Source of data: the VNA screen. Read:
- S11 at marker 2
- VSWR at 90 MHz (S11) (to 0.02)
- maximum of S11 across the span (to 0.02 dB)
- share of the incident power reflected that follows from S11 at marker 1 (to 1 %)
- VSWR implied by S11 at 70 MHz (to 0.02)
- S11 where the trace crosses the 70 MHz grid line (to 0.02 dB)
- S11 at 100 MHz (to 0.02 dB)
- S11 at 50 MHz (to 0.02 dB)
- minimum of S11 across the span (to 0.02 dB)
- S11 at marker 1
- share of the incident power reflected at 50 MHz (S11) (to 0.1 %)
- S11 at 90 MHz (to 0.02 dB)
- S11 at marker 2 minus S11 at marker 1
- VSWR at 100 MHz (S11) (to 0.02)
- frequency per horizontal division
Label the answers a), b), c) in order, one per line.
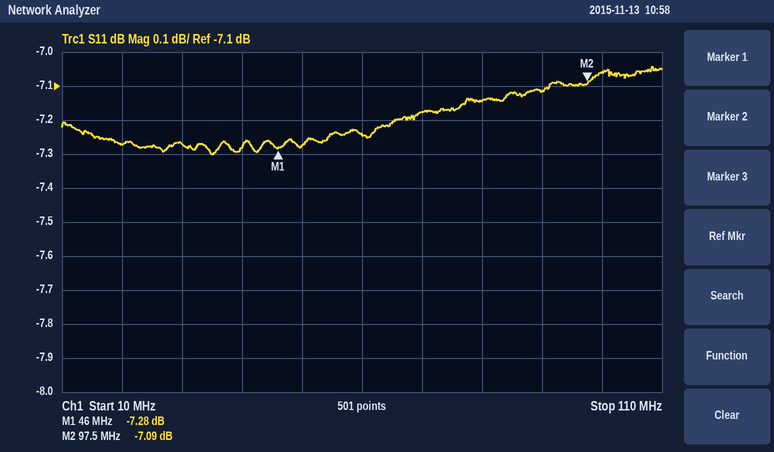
a) -7.09 dB
b) 2.58
c) -7.04 dB
d) 19 %
e) 2.56
f) -7.18 dB
g) -7.06 dB
h) -7.28 dB
i) -7.30 dB
j) -7.28 dB
k) 18.7 %
l) -7.12 dB
m) 0.19 dB
n) 2.60
o) 10 MHz
